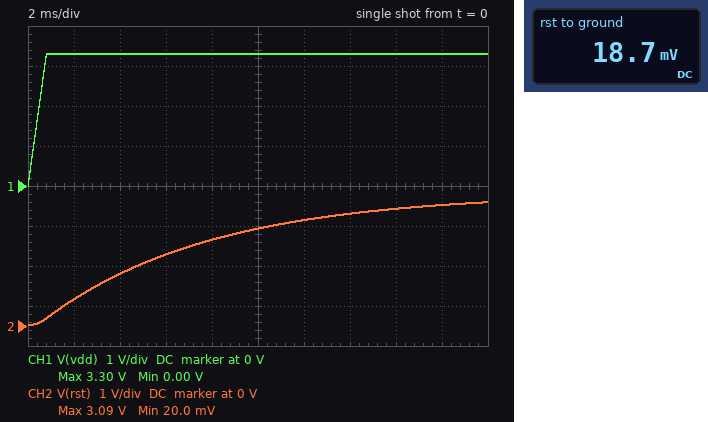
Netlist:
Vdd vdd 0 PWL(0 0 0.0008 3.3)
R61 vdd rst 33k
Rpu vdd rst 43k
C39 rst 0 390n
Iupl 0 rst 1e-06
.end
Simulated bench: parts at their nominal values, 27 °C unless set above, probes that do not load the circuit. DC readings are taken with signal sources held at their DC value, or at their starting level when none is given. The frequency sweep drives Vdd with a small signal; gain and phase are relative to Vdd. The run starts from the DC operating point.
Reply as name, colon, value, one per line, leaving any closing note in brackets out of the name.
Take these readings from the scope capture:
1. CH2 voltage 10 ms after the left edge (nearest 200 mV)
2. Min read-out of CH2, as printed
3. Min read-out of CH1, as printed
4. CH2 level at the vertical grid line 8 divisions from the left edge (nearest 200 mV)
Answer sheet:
CH2 voltage 10 ms after the left edge: 2.4 V
Min read-out of CH2, as printed: 20.0 mV
Min read-out of CH1, as printed: 0.00 V
CH2 level at the vertical grid line 8 divisions from the left edge: 3.0 V
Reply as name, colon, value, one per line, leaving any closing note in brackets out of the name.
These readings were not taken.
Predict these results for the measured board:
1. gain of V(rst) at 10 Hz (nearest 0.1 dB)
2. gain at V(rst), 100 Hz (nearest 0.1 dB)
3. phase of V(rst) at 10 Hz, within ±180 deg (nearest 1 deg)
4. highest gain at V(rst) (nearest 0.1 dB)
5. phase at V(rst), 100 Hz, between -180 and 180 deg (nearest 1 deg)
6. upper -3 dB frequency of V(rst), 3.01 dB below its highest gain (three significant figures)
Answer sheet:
gain of V(rst) at 10 Hz: -0.8 dB
gain at V(rst), 100 Hz: -13.4 dB
phase of V(rst) at 10 Hz, within ±180 deg: -25 deg
highest gain at V(rst): 0 dB
phase at V(rst), 100 Hz, between -180 and 180 deg: -78 deg
upper -3 dB frequency of V(rst), 3.01 dB below its highest gain: 21.9 Hz
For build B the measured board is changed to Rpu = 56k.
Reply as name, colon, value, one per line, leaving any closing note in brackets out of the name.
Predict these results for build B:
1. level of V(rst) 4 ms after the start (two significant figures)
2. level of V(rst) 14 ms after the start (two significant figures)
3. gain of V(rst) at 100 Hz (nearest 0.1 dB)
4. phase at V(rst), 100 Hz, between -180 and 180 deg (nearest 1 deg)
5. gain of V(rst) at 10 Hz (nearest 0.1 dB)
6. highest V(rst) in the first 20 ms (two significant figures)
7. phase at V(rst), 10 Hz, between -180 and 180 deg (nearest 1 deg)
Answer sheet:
level of V(rst) 4 ms after the start: 1.2 V
level of V(rst) 14 ms after the start: 2.7 V
gain of V(rst) at 100 Hz: -14.3 dB
phase at V(rst), 100 Hz, between -180 and 180 deg: -79 deg
gain of V(rst) at 10 Hz: -1.0 dB
highest V(rst) in the first 20 ms: 3.0 V
phase at V(rst), 10 Hz, between -180 and 180 deg: -27 deg
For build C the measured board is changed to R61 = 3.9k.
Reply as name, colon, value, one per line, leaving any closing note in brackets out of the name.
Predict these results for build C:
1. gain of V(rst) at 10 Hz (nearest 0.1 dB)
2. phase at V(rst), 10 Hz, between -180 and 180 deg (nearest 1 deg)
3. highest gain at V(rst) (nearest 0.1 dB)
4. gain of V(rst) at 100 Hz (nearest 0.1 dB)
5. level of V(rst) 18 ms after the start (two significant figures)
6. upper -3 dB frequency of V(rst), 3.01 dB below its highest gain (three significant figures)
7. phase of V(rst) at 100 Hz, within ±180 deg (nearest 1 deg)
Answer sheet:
gain of V(rst) at 10 Hz: 0 dB
phase at V(rst), 10 Hz, between -180 and 180 deg: -5 deg
highest gain at V(rst): 0 dB
gain of V(rst) at 100 Hz: -2.5 dB
level of V(rst) 18 ms after the start: 3.3 V
upper -3 dB frequency of V(rst), 3.01 dB below its highest gain: 114 Hz
phase of V(rst) at 100 Hz, within ±180 deg: -41 deg
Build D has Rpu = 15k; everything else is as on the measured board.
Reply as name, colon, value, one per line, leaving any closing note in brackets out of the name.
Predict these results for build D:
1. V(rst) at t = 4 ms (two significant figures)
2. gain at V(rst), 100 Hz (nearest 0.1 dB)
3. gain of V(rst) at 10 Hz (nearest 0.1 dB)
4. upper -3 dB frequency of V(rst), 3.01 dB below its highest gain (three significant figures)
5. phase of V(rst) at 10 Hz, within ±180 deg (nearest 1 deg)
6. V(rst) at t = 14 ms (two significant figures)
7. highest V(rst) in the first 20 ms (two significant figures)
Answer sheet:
V(rst) at t = 4 ms: 2.0 V
gain at V(rst), 100 Hz: -8.7 dB
gain of V(rst) at 10 Hz: -0.3 dB
upper -3 dB frequency of V(rst), 3.01 dB below its highest gain: 39.6 Hz
phase of V(rst) at 10 Hz, within ±180 deg: -14 deg
V(rst) at t = 14 ms: 3.2 V
highest V(rst) in the first 20 ms: 3.3 V
